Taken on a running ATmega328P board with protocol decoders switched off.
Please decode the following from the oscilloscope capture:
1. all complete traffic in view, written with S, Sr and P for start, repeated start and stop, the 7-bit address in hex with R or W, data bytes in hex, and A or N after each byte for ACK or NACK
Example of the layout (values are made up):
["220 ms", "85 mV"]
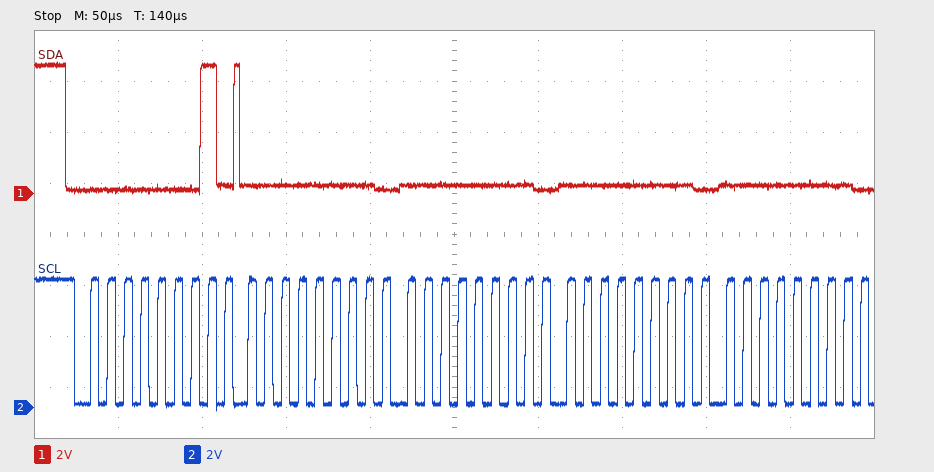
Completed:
["S 00R A 00 A 00 A 00 A 00 A"]
